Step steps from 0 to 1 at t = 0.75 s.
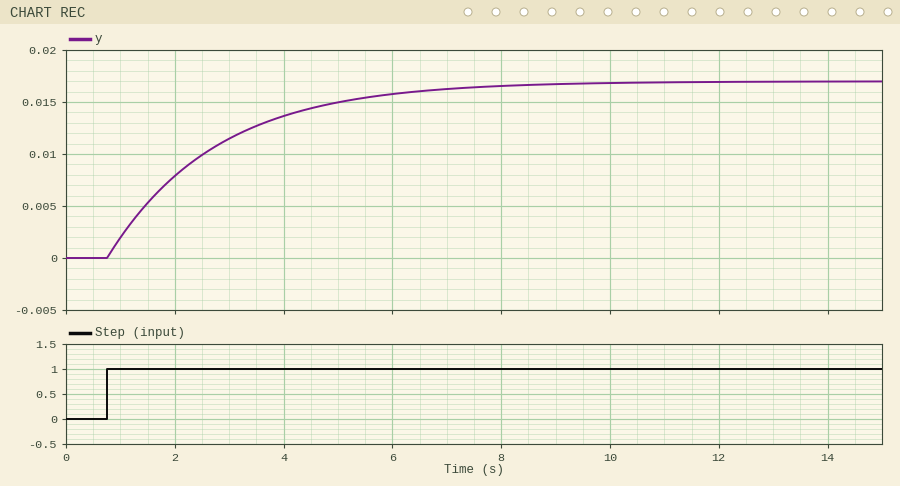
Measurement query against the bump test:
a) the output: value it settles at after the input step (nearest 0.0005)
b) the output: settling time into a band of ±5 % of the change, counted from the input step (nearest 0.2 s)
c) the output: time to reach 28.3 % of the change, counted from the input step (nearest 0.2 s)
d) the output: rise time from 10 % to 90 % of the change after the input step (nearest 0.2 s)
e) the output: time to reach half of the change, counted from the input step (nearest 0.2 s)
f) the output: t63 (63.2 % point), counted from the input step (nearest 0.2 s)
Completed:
0.0170
6.0 s
0.6 s
4.4 s
1.4 s
2.0 s
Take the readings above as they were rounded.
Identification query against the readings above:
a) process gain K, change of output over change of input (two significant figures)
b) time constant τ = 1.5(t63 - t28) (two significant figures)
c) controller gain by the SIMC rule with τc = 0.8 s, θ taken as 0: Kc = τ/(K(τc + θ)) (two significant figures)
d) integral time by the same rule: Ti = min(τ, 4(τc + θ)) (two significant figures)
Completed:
0.017
2.1 s
150
2.1 s
